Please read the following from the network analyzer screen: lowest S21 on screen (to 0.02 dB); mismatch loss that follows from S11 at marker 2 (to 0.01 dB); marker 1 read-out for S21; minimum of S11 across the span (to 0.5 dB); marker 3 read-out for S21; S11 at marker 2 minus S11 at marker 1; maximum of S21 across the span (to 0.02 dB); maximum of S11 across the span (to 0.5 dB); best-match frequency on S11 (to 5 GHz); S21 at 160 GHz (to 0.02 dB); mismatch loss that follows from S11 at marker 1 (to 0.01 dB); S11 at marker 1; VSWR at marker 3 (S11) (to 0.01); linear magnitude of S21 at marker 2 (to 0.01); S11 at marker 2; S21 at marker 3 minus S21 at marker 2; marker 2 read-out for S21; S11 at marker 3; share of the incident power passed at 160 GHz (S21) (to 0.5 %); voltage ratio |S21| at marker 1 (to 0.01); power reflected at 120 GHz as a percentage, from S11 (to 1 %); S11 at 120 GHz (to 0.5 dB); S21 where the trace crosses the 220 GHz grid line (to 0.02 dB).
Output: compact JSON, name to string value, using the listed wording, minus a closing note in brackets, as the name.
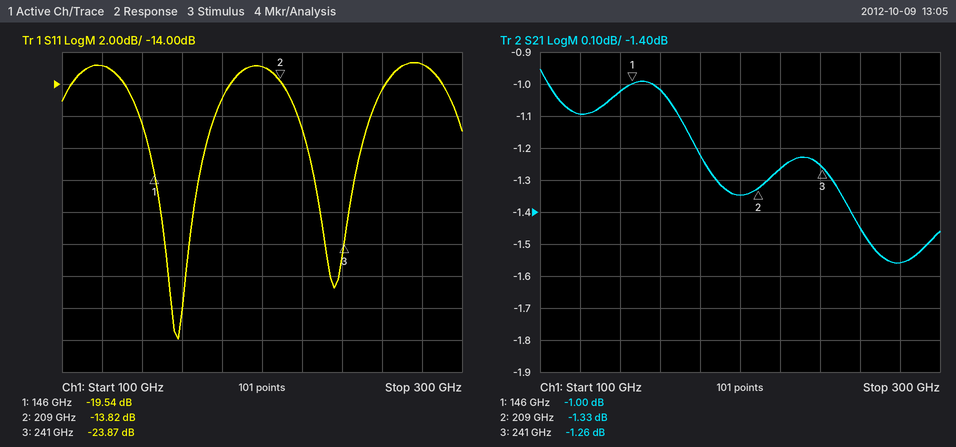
{"lowest S21 on screen": "-1.56 dB", "mismatch loss that follows from S11 at marker 2": "0.18 dB", "marker 1 read-out for S21": "-1.00 dB", "minimum of S11 across the span": "-30.0 dB", "marker 3 read-out for S21": "-1.26 dB", "S11 at marker 2 minus S11 at marker 1": "5.72 dB", "maximum of S21 across the span": "-0.96 dB", "maximum of S11 across the span": "-12.5 dB", "best-match frequency on S11": "160 GHz", "S21 at 160 GHz": "-1.02 dB", "mismatch loss that follows from S11 at marker 1": "0.05 dB", "S11 at marker 1": "-19.54 dB", "VSWR at marker 3 (S11)": "1.14", "linear magnitude of S21 at marker 2": "0.86", "S11 at marker 2": "-13.82 dB", "S21 at marker 3 minus S21 at marker 2": "0.07 dB", "marker 2 read-out for S21": "-1.33 dB", "S11 at marker 3": "-23.87 dB", "share of the incident power passed at 160 GHz (S21)": "79.0 %", "voltage ratio |S21| at marker 1": "0.89", "power reflected at 120 GHz as a percentage, from S11": "5 %", "S11 at 120 GHz": "-13.0 dB", "S21 where the trace crosses the 220 GHz grid line": "-1.26 dB"}
